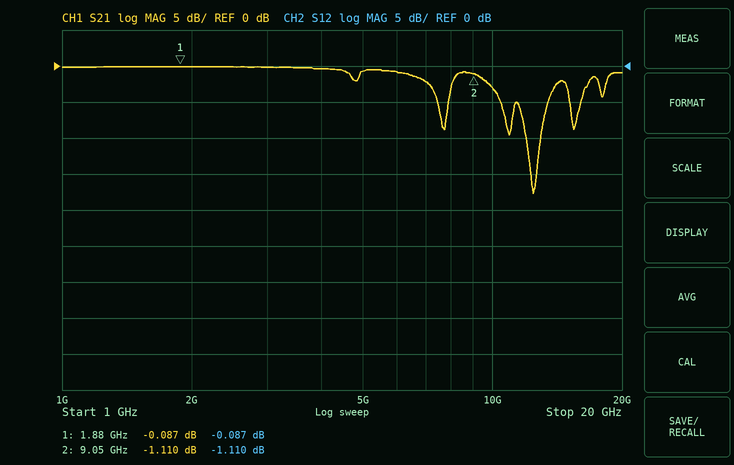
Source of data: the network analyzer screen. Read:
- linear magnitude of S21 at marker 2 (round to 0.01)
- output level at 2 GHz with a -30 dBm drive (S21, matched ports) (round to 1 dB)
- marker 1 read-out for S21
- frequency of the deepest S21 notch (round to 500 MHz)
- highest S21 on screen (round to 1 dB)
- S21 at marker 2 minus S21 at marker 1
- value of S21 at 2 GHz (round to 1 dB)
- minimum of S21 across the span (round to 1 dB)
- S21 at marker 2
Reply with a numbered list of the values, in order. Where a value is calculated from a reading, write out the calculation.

1. 10^(-1.11/20) ≈ 0.88
2. -30 dBm + (0 dB) = -30 dBm
3. -0.087 dB
4. 12.5 GHz
5. 0 dB
6. -1.11 − (-0.087) = -1.023 dB
7. 0 dB
8. -18 dB
9. -1.110 dB
